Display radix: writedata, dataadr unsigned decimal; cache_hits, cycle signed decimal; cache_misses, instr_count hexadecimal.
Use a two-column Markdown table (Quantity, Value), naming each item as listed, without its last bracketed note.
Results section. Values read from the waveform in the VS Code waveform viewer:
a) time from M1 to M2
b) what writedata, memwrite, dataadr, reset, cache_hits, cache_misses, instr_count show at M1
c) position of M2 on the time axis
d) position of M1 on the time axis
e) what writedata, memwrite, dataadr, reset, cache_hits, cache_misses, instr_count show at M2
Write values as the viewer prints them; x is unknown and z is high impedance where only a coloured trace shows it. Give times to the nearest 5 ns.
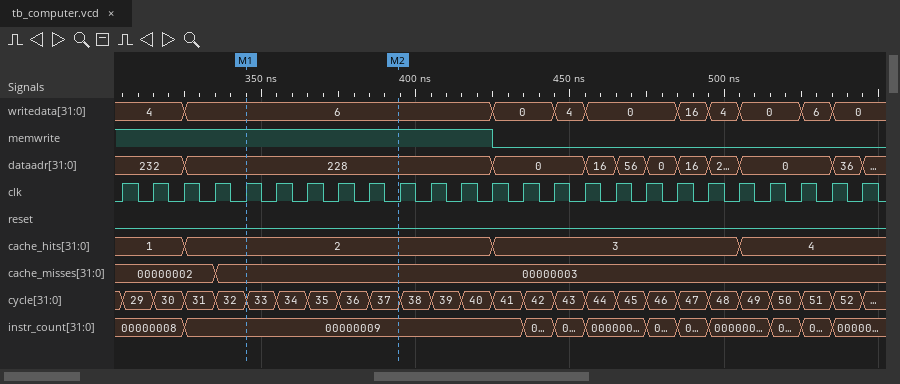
| Quantity | Value |
|---|---|
| time from M1 to M2 | 50 ns |
| what writedata, memwrite, dataadr, reset, cache_hits, cache_misses, instr_count show at M1 | writedata=6, memwrite=1, dataadr=228, reset=0, cache_hits=2, cache_misses=00000003, instr_count=00000009 |
| position of M2 on the time axis | 395 ns |
| position of M1 on the time axis | 345 ns |
| what writedata, memwrite, dataadr, reset, cache_hits, cache_misses, instr_count show at M2 | writedata=6, memwrite=1, dataadr=228, reset=0, cache_hits=2, cache_misses=00000003, instr_count=00000009 |
